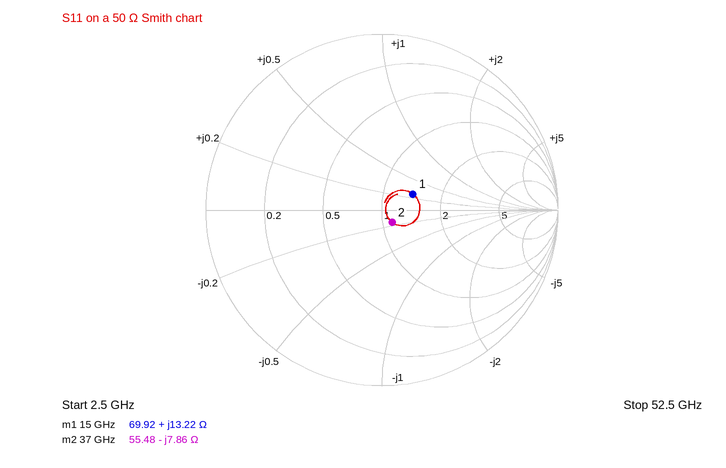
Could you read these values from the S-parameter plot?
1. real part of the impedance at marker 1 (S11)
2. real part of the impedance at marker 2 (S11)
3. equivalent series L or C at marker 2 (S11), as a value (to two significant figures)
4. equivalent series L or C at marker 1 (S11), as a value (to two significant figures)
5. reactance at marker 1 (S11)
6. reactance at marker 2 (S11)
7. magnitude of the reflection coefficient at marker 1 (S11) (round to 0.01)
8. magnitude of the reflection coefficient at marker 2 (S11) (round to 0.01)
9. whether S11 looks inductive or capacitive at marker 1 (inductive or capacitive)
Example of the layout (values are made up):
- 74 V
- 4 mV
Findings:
- 69.92 Ω
- 55.48 Ω
- 550 fF
- 140 pH
- +13.22 Ω
- -7.86 Ω
- 0.20
- 0.09
- inductive
